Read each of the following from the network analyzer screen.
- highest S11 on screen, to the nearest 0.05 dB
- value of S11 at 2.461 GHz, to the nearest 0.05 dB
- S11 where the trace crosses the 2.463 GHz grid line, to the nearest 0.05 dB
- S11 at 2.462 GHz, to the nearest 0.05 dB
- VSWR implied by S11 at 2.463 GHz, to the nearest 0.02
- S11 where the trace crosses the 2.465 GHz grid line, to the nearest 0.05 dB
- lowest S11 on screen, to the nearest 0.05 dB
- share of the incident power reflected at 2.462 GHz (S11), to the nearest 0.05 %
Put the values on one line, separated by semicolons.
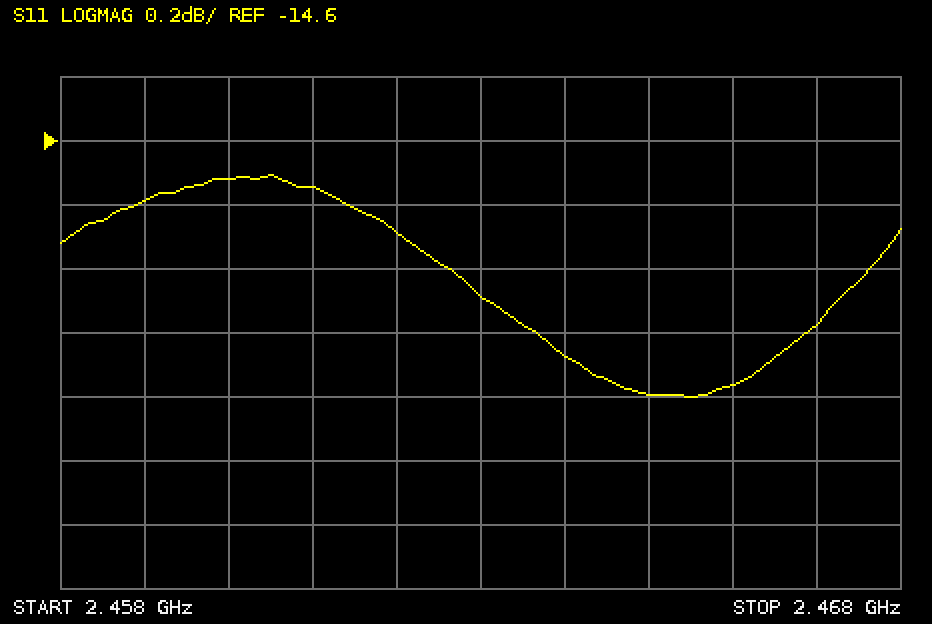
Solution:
-14.70 dB; -14.75 dB; -15.10 dB; -14.90 dB; 1.42; -15.40 dB; -15.40 dB; 3.25 %
